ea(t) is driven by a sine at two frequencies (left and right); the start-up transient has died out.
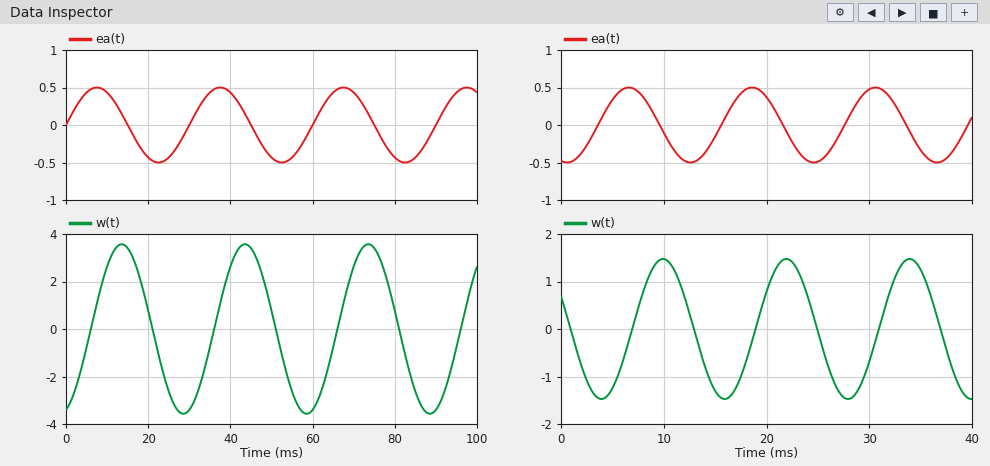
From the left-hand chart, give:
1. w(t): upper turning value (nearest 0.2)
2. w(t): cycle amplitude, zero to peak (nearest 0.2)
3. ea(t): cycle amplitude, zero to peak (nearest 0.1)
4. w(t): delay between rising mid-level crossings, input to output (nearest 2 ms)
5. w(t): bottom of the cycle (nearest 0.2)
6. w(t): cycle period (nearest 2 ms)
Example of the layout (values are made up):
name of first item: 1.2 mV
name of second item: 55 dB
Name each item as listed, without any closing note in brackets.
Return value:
w(t): upper turning value: 3.6
w(t): cycle amplitude, zero to peak: 3.6
ea(t): cycle amplitude, zero to peak: 0.5
w(t): delay between rising mid-level crossings, input to output: 6 ms
w(t): bottom of the cycle: -3.6
w(t): cycle period: 30 ms
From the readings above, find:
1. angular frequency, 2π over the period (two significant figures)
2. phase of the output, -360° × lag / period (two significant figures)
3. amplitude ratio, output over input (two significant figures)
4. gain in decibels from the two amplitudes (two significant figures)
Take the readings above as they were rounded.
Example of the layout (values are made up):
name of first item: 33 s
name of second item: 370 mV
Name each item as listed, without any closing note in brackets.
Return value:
angular frequency, 2π over the period: 0.21 rad/ms
phase of the output, -360° × lag / period: -72°
amplitude ratio, output over input: 7.2
gain in decibels from the two amplitudes: 17 dB
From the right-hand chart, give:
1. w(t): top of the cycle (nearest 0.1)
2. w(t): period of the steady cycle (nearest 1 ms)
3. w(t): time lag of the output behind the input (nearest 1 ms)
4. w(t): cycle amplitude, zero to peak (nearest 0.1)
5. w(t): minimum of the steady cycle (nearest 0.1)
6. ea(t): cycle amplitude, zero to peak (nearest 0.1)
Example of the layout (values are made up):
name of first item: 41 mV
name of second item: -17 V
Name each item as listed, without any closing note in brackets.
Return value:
w(t): top of the cycle: 1.5
w(t): period of the steady cycle: 12 ms
w(t): time lag of the output behind the input: 3 ms
w(t): cycle amplitude, zero to peak: 1.5
w(t): minimum of the steady cycle: -1.5
ea(t): cycle amplitude, zero to peak: 0.5
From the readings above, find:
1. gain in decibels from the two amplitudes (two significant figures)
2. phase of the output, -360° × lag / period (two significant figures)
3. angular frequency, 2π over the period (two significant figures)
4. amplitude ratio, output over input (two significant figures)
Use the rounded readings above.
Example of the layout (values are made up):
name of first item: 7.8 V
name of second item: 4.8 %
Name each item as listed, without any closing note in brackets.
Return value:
gain in decibels from the two amplitudes: 9.5 dB
phase of the output, -360° × lag / period: -90°
angular frequency, 2π over the period: 0.52 rad/ms
amplitude ratio, output over input: 3.0
